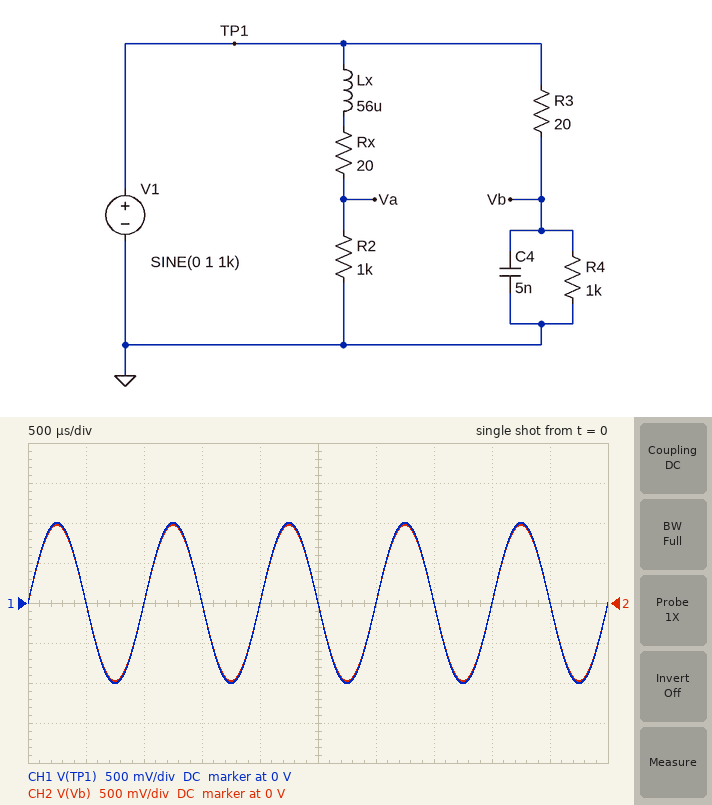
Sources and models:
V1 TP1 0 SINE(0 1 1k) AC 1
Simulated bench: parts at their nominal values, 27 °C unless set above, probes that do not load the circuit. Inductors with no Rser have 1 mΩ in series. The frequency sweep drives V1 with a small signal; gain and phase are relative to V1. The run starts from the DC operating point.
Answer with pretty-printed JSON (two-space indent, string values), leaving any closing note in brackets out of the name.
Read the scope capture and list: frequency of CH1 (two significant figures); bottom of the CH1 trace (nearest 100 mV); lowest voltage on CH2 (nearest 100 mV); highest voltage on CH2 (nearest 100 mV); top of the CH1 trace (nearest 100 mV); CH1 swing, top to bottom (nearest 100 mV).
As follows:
{
  "frequency of CH1": "1.0 kHz",
  "bottom of the CH1 trace": "-1.0 V",
  "lowest voltage on CH2": "-1.0 V",
  "highest voltage on CH2": "1.0 V",
  "top of the CH1 trace": "1.0 V",
  "CH1 swing, top to bottom": "2.0 V"
}
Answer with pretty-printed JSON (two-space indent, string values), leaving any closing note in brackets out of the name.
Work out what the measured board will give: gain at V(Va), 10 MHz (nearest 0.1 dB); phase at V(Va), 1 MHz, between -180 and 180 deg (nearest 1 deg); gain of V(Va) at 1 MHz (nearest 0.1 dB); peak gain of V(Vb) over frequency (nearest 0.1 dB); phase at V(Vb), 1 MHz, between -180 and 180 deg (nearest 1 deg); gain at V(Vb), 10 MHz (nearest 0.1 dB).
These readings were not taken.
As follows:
{
  "gain at V(Va), 10 MHz": "-11.3 dB",
  "phase at V(Va), 1 MHz, between -180 and 180 deg": "-19 deg",
  "gain of V(Va) at 1 MHz": "-0.7 dB",
  "peak gain of V(Vb) over frequency": "-0.2 dB",
  "phase at V(Vb), 1 MHz, between -180 and 180 deg": "-32 deg",
  "gain at V(Vb), 10 MHz": "-16.1 dB"
}
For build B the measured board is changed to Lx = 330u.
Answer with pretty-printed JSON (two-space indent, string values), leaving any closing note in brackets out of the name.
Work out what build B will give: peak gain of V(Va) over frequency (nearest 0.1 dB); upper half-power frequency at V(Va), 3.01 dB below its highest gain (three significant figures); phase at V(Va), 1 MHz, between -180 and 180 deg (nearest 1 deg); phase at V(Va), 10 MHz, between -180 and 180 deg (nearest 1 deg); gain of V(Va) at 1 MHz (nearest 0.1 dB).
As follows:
{
  "peak gain of V(Va) over frequency": "-0.2 dB",
  "upper half-power frequency at V(Va), 3.01 dB below its highest gain": "492 kHz",
  "phase at V(Va), 1 MHz, between -180 and 180 deg": "-64 deg",
  "phase at V(Va), 10 MHz, between -180 and 180 deg": "-87 deg",
  "gain of V(Va) at 1 MHz": "-7.3 dB"
}
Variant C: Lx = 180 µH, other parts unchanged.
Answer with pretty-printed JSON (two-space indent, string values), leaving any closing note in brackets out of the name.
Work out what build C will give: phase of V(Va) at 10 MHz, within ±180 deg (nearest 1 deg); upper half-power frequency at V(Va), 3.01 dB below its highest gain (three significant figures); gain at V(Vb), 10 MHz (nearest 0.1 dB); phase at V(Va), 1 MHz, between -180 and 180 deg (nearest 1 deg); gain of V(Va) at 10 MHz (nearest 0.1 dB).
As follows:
{
  "phase of V(Va) at 10 MHz, within ±180 deg": "-85 deg",
  "upper half-power frequency at V(Va), 3.01 dB below its highest gain": "902 kHz",
  "gain at V(Vb), 10 MHz": "-16.1 dB",
  "phase at V(Va), 1 MHz, between -180 and 180 deg": "-48 deg",
  "gain of V(Va) at 10 MHz": "-21.1 dB"
}
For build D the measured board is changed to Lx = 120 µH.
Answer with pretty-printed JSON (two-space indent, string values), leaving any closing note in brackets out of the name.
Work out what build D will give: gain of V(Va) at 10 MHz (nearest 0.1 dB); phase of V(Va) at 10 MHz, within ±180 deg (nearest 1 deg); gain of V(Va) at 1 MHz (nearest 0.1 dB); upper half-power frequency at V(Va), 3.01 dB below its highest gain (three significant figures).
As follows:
{
  "gain of V(Va) at 10 MHz": "-17.6 dB",
  "phase of V(Va) at 10 MHz, within ±180 deg": "-82 deg",
  "gain of V(Va) at 1 MHz": "-2.1 dB",
  "upper half-power frequency at V(Va), 3.01 dB below its highest gain": "1.35 MHz"
}
